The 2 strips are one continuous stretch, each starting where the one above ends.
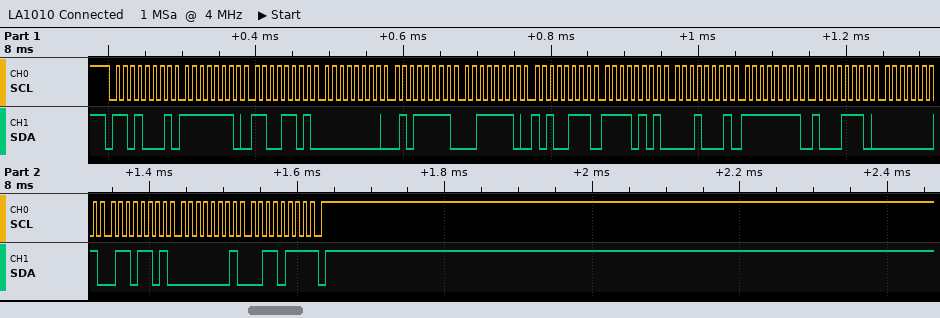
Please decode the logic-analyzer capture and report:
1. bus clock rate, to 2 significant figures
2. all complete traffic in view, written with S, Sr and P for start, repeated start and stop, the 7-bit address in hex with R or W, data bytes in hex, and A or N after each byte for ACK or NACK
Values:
100 kHz
S 68R A FE A CD A 00 A 5F A 3E A A7 A F5 A 11 A FF A 8E A 01 A 6D A 01 A 37 N P
